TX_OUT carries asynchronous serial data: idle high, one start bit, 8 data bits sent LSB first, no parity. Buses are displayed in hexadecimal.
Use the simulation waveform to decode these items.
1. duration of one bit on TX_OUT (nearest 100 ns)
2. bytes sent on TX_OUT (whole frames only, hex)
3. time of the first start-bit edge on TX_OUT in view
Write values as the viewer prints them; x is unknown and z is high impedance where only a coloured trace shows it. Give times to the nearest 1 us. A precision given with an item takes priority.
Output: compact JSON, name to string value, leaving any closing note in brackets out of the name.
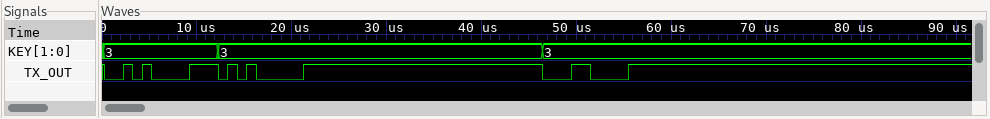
{"duration of one bit on TX_OUT": "1000 ns", "bytes sent on TX_OUT": "0A, 05, 0C", "time of the first start-bit edge on TX_OUT in view": "0 us"}
